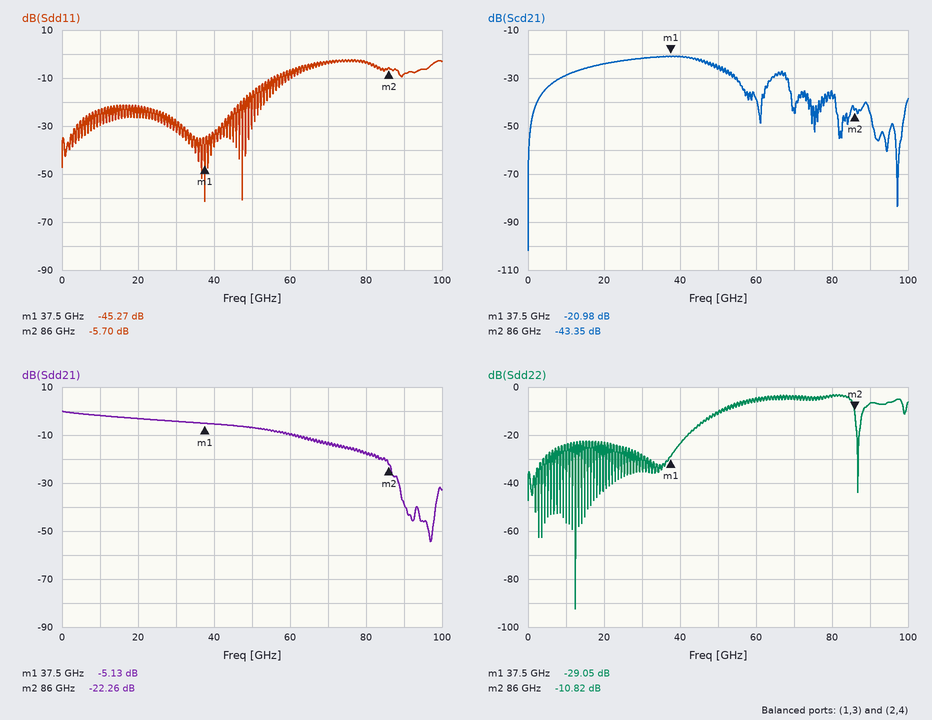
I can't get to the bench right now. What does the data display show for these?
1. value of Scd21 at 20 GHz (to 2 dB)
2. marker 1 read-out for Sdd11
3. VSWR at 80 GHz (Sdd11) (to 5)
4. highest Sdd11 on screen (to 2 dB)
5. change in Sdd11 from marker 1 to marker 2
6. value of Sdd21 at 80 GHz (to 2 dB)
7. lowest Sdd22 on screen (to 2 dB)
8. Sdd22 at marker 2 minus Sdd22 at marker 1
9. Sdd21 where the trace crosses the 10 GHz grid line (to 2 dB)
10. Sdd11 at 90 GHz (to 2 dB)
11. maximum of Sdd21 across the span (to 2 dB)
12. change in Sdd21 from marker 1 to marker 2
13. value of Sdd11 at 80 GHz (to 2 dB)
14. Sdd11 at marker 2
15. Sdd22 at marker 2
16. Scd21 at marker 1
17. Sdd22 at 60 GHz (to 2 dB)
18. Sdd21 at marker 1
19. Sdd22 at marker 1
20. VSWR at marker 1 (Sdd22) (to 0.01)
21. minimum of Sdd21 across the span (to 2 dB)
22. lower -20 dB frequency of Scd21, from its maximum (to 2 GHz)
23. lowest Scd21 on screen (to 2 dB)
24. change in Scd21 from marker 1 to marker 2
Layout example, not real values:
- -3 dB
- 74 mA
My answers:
- -24 dB
- -45.27 dB
- 5
- -2 dB
- 39.57 dB
- -18 dB
- -92 dB
- 18.23 dB
- -2 dB
- -8 dB
- 0 dB
- -17.13 dB
- -4 dB
- -5.70 dB
- -10.82 dB
- -20.98 dB
- -4 dB
- -5.13 dB
- -29.05 dB
- 1.07
- -54 dB
- 2 GHz
- -102 dB
- -22.37 dB
